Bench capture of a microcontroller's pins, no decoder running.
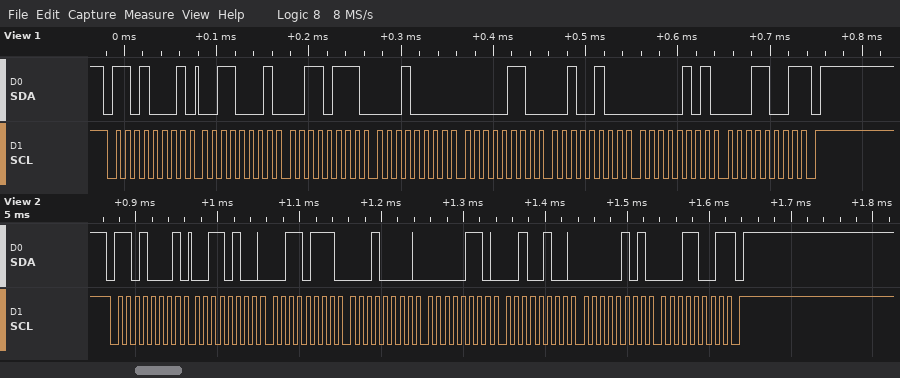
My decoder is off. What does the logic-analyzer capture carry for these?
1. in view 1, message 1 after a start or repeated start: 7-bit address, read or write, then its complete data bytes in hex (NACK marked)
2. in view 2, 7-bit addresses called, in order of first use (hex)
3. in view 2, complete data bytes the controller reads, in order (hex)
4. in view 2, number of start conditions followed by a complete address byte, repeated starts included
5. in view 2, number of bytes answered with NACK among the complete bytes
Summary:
0x68 read: 31 37 10 06 24 05 19 NACK
0x68
34 37 10 06 24 05 19
1
1
